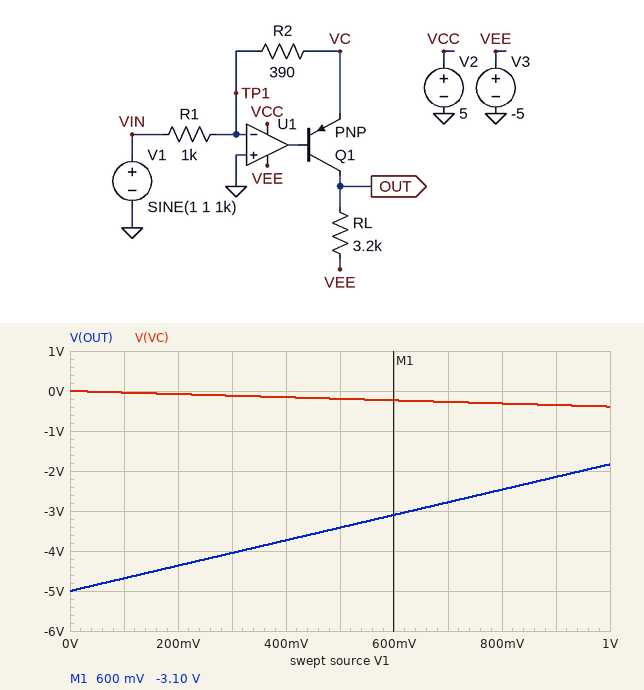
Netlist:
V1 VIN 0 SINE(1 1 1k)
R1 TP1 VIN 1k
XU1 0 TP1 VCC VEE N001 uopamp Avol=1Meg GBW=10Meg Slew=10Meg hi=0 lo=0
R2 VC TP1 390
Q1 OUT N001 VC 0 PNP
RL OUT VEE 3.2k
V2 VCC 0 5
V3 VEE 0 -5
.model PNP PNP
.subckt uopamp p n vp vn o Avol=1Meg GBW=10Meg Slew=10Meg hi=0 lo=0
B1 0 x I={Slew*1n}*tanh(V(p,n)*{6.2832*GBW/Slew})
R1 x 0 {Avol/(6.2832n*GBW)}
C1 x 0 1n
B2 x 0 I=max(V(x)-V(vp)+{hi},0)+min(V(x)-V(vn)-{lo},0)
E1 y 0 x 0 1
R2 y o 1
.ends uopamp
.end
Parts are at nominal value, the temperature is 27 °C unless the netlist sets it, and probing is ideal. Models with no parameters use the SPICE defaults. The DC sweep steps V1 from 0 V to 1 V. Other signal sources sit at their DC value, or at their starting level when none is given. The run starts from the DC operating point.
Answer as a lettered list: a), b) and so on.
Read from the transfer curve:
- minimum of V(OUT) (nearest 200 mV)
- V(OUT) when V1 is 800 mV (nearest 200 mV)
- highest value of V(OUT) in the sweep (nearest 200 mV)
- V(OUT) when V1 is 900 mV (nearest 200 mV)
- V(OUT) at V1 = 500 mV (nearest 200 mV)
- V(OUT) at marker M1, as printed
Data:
a) -5.0 V
b) -2.4 V
c) -1.8 V
d) -2.2 V
e) -3.4 V
f) -3.10 V
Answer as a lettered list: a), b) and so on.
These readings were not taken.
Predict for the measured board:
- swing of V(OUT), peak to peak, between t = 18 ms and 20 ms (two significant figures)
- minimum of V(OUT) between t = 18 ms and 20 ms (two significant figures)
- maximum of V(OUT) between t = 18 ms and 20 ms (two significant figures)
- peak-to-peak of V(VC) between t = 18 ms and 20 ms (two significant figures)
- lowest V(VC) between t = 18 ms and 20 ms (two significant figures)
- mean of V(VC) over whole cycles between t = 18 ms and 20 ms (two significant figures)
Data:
a) 4.4 V
b) -5.0 V
c) -640 mV
d) 780 mV
e) -780 mV
f) -390 mV
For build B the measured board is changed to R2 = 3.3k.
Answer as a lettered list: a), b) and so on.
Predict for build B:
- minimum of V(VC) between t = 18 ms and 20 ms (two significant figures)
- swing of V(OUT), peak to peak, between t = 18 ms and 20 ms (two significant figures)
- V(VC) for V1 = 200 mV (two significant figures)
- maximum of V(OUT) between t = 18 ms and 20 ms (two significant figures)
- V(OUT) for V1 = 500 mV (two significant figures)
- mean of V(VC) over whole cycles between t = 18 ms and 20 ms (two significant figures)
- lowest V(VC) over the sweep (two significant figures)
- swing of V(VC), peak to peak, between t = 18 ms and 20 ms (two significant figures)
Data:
a) -4.2 V
b) 2.4 V
c) -660 mV
d) -2.6 V
e) -3.4 V
f) -2.7 V
g) -3.3 V
h) 4.2 V
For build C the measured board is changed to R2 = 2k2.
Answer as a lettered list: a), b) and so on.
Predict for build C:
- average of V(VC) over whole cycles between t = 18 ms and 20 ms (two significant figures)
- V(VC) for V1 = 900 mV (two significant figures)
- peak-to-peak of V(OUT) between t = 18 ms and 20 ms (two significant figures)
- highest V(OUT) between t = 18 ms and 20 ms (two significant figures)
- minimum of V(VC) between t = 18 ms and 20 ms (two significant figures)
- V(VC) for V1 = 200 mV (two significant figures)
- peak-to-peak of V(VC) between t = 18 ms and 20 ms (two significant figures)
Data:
a) -2.2 V
b) -2.0 V
c) 2.9 V
d) -2.1 V
e) -4.2 V
f) -440 mV
g) 4.2 V
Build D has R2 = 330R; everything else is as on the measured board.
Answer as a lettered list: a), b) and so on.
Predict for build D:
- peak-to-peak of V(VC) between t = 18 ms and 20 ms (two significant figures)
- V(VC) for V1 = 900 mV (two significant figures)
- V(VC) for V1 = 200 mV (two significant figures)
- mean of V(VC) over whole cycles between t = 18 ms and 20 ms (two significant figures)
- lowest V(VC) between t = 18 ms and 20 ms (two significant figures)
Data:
a) 660 mV
b) -300 mV
c) -66 mV
d) -330 mV
e) -660 mV
